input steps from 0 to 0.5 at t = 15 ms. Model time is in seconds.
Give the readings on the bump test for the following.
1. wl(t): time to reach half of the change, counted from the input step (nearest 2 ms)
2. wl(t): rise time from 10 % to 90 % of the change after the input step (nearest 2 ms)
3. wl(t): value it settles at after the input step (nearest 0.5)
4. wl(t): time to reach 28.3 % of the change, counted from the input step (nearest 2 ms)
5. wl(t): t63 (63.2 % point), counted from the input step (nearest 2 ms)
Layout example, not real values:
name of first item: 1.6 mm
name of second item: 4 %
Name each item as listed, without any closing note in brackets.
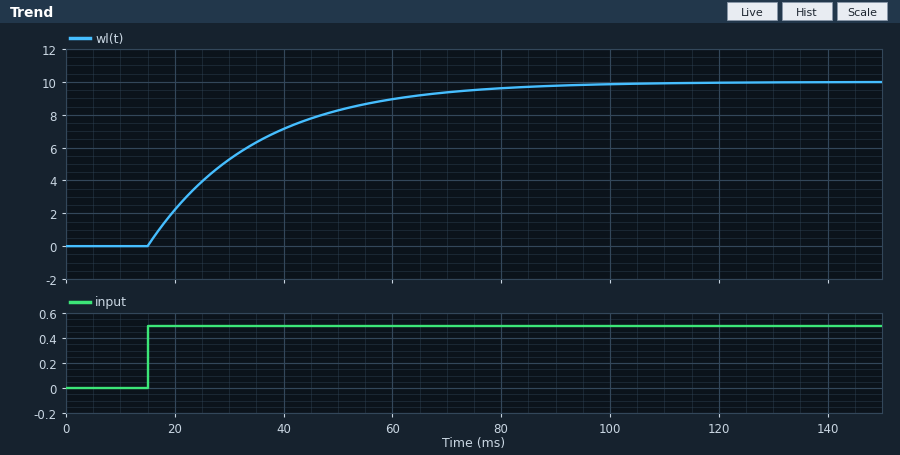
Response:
wl(t): time to reach half of the change, counted from the input step: 14 ms
wl(t): rise time from 10 % to 90 % of the change after the input step: 44 ms
wl(t): value it settles at after the input step: 10.0
wl(t): time to reach 28.3 % of the change, counted from the input step: 6 ms
wl(t): t63 (63.2 % point), counted from the input step: 20 ms
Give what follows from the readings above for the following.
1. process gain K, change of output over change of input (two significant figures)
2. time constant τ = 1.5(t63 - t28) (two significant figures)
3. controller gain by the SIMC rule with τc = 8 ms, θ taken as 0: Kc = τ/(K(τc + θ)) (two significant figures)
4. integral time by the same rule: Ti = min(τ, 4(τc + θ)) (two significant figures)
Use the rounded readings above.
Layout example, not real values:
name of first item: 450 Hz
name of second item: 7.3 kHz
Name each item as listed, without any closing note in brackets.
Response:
process gain K, change of output over change of input: 20
time constant τ = 1.5(t63 - t28): 21 ms
controller gain by the SIMC rule with τc = 8 ms, θ taken as 0: Kc = τ/(K(τc + θ)): 0.13
integral time by the same rule: Ti = min(τ, 4(τc + θ)): 21 ms
